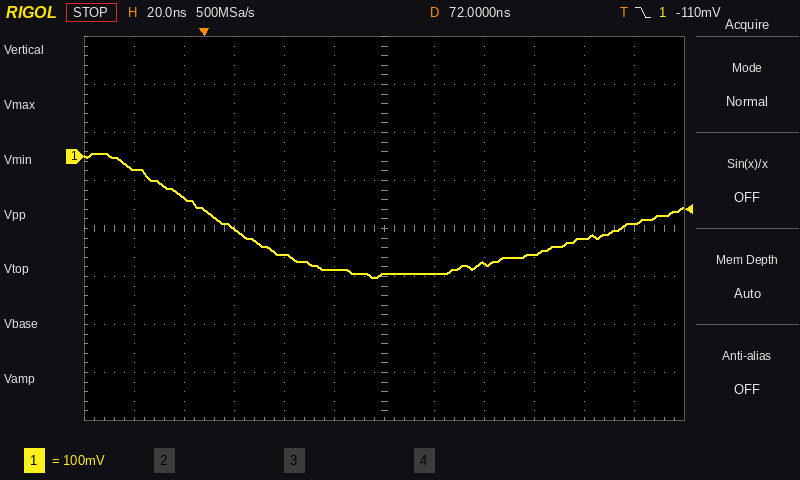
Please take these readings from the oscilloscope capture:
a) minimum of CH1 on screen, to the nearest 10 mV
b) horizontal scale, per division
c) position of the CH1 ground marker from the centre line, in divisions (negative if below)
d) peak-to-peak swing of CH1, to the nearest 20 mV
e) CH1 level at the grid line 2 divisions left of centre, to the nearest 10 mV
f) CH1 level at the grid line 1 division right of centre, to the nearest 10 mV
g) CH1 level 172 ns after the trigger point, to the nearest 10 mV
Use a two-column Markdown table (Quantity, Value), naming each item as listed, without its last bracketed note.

| Quantity | Value |
|---|---|
| minimum of CH1 on screen, to the nearest 10 mV | -250 mV |
| horizontal scale, per division | 20 ns |
| position of the CH1 ground marker from the centre line, in divisions | +1.5 div |
| peak-to-peak swing of CH1, to the nearest 20 mV | 260 mV |
| CH1 level at the grid line 2 divisions left of centre, to the nearest 10 mV | -200 mV |
| CH1 level at the grid line 1 division right of centre, to the nearest 10 mV | -240 mV |
| CH1 level 172 ns after the trigger point, to the nearest 10 mV | -140 mV |
